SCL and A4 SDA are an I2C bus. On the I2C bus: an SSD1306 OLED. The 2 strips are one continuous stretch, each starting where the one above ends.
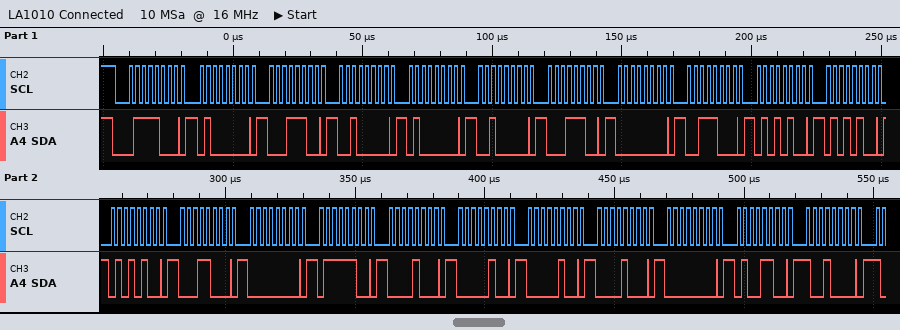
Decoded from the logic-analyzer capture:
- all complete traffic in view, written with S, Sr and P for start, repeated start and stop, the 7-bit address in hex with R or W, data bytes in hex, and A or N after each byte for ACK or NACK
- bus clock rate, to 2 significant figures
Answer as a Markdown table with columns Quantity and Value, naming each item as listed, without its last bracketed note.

| Quantity | Value |
|---|---|
| all complete traffic in view, written with S, Sr and P for start, repeated start and stop, the 7-bit address in hex with R or W, data bytes in hex, and A or N after each byte for ACK or NACK | S 3CW A 40 A 1C A 20 A 40 A 20 A 1C A 00 A 38 A 54 A 54 A 54 A 18 A 00 A 7C A 08 A 04 A 04 A 08 A 00 A 4C A 90 A |
| bus clock rate, to 2 significant figures | 400 kHz |
